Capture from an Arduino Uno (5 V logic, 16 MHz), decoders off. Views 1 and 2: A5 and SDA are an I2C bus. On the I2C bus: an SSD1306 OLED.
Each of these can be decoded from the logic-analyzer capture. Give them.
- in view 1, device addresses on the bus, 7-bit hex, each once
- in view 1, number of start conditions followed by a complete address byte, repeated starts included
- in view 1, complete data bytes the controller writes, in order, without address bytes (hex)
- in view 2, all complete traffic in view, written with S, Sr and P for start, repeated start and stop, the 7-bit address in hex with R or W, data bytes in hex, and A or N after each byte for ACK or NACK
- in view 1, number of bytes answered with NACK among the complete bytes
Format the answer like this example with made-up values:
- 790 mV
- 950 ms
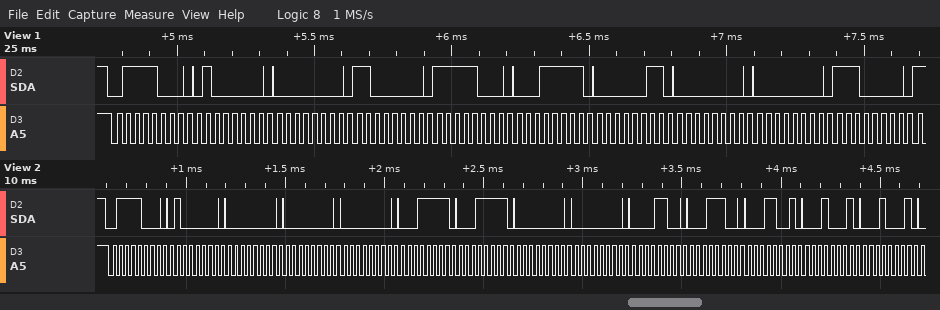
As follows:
- 0x3C
- 1
- 40 00 C0 F8 1F 03 00 00 E0
- S 3CW A 40 A 00 A 00 A 00 A 1F A 1F A 00 A 00 A 0C A 1C A 19 A 11 A 11 A
- 0
